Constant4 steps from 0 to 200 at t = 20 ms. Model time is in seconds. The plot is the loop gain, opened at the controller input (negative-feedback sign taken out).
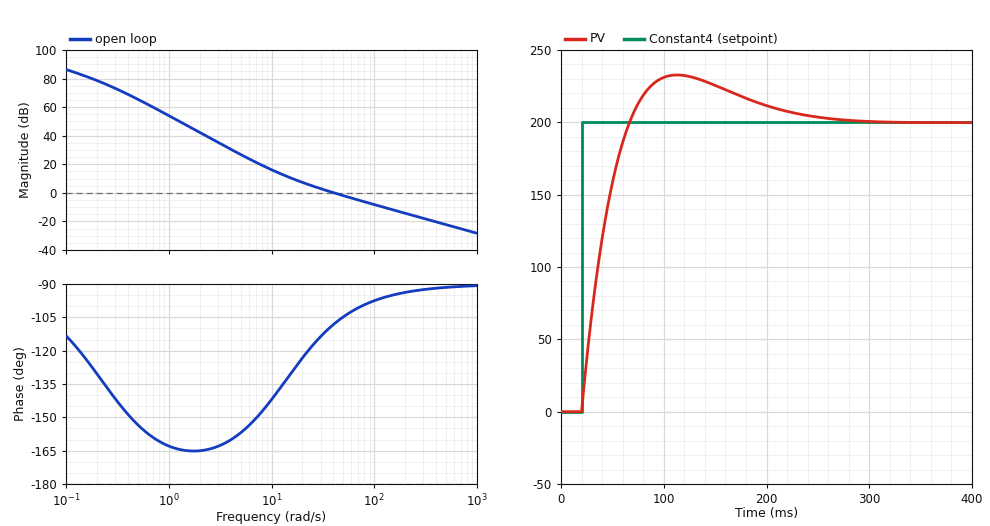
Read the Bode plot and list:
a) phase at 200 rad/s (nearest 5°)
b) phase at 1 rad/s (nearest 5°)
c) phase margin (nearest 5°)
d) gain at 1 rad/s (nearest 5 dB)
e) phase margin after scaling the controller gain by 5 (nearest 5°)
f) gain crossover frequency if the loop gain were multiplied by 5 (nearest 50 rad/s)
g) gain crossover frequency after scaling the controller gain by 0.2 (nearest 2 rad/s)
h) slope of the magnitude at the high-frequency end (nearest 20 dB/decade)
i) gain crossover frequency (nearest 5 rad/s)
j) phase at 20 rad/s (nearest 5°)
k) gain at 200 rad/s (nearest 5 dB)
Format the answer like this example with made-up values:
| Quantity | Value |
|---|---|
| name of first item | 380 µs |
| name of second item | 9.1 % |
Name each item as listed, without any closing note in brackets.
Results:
| Quantity | Value |
|---|---|
| phase at 200 rad/s | -95° |
| phase at 1 rad/s | -165° |
| phase margin | 70° |
| gain at 1 rad/s | 55 dB |
| phase margin after scaling the controller gain by 5 | 85° |
| gain crossover frequency if the loop gain were multiplied by 5 | 200 rad/s |
| gain crossover frequency after scaling the controller gain by 0.2 | 12 rad/s |
| slope of the magnitude at the high-frequency end | -20 dB/decade |
| gain crossover frequency | 40 rad/s |
| phase at 20 rad/s | -125° |
| gain at 200 rad/s | -15 dB |
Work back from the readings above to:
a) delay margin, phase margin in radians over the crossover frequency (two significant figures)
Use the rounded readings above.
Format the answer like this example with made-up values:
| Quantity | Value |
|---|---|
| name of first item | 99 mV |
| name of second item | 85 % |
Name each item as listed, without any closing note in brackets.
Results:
| Quantity | Value |
|---|---|
| delay margin, phase margin in radians over the crossover frequency | 0.031 s |
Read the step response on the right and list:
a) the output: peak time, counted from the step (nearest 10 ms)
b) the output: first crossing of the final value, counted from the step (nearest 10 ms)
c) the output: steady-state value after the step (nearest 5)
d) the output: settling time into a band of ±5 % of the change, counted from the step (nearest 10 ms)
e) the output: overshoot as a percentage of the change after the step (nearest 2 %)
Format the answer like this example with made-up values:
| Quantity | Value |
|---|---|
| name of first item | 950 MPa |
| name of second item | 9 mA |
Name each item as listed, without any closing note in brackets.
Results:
| Quantity | Value |
|---|---|
| the output: peak time, counted from the step | 90 ms |
| the output: first crossing of the final value, counted from the step | 50 ms |
| the output: steady-state value after the step | 200 |
| the output: settling time into a band of ±5 % of the change, counted from the step | 190 ms |
| the output: overshoot as a percentage of the change after the step | 16 % |
